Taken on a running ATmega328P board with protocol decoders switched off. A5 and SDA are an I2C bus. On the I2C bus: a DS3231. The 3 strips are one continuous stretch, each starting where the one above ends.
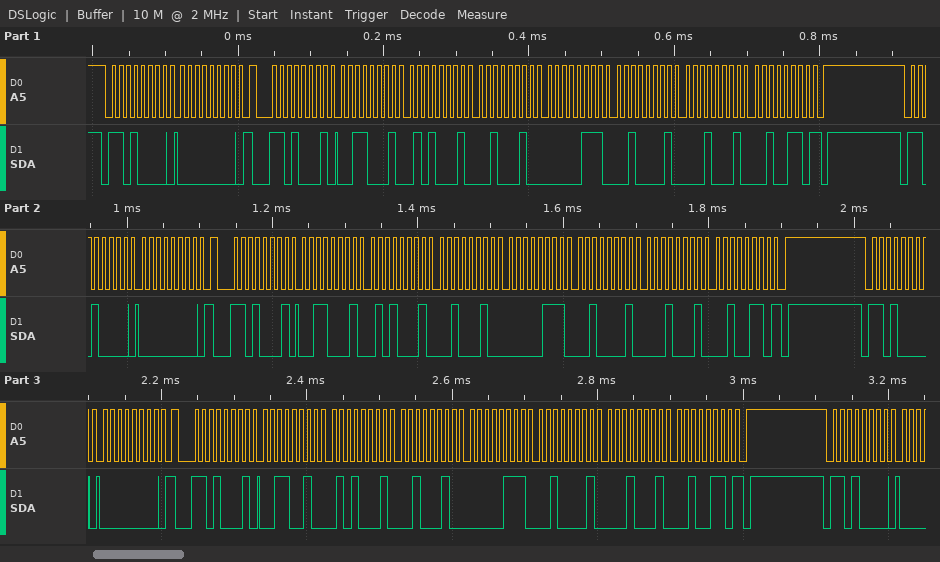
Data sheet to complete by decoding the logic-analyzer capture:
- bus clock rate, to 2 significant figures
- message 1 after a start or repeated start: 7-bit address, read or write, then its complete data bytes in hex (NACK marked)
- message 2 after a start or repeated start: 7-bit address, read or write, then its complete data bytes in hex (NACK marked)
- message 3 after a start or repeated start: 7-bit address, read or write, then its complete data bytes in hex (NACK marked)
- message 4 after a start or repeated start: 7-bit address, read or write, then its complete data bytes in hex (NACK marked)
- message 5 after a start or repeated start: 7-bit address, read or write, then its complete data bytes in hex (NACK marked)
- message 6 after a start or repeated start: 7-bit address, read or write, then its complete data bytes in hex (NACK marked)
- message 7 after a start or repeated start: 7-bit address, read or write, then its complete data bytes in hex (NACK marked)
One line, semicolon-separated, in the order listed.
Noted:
100 kHz; 0x68 write: 00; 0x68 read: 31 51 22 07 21 11 26 NACK; 0x68 write: 00; 0x68 read: 31 51 22 07 21 11 26 NACK; 0x68 write: 00; 0x68 read: 32 51 22 07 21 11 26 NACK; 0x68 write
